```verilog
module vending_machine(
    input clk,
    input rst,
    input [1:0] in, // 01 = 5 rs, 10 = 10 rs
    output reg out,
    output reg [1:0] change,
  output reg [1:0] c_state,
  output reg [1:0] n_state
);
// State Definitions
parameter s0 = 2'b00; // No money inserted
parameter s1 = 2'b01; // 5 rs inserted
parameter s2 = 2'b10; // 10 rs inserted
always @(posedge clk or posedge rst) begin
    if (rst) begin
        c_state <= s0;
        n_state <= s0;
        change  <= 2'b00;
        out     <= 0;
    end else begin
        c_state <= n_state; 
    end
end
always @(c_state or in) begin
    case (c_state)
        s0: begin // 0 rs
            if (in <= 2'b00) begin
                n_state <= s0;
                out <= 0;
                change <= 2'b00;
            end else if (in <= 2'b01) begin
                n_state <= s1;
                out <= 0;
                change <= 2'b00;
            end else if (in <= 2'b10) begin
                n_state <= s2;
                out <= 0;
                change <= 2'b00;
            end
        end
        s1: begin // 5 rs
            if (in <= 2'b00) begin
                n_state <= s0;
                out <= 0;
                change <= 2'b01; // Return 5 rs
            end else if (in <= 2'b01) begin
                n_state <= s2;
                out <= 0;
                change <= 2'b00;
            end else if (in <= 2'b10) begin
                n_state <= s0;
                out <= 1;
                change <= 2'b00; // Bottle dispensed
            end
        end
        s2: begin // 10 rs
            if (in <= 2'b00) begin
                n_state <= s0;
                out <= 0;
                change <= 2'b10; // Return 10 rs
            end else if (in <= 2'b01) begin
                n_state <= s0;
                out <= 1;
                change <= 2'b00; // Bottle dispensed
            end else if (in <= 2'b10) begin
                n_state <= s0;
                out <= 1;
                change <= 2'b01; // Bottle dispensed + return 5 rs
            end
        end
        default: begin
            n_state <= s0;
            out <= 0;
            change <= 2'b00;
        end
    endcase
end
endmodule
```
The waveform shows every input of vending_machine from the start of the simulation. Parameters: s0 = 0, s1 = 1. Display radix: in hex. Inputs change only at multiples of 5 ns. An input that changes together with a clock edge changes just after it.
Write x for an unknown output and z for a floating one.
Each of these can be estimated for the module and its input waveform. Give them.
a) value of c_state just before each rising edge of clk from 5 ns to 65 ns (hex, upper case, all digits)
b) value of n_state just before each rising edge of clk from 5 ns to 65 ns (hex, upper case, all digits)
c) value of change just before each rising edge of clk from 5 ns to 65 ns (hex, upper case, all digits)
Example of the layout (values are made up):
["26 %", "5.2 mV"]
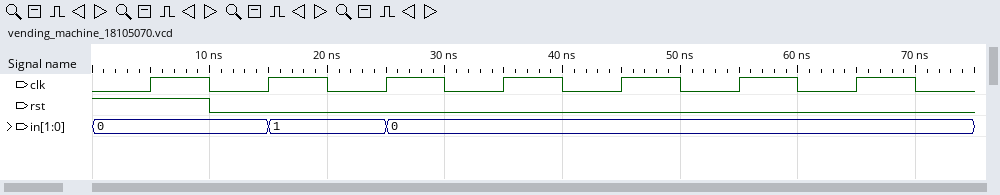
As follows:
["0, 0, 0, 1, 0, 0, 0", "0, 0, 1, 0, 0, 0, 0", "0, 0, 0, 1, 0, 0, 0"]
